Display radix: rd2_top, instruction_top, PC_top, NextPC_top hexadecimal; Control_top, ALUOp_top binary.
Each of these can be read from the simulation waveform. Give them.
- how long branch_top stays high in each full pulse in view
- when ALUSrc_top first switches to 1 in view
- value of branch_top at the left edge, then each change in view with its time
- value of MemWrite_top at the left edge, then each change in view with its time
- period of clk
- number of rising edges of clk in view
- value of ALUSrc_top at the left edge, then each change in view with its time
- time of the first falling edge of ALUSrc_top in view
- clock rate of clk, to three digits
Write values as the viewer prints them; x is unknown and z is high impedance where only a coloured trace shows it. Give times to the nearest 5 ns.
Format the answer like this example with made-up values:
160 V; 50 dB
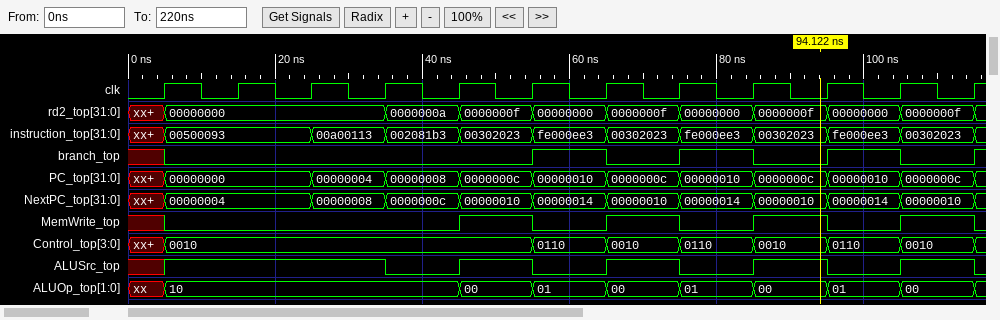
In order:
10 ns, 10 ns, 10 ns; 5 ns; x, 0 at 5 ns, 1 at 55 ns, 0 at 65 ns, 1 at 75 ns, 0 at 85 ns, 1 at 95 ns, 0 at 105 ns, 1 at 115 ns; x, 0 at 5 ns, 1 at 45 ns, 0 at 55 ns, 1 at 65 ns, 0 at 75 ns, 1 at 85 ns, 0 at 95 ns, 1 at 105 ns, 0 at 115 ns; 10 ns; 12; x, 1 at 5 ns, 0 at 35 ns, 1 at 45 ns, 0 at 55 ns, 1 at 65 ns, 0 at 75 ns, 1 at 85 ns, 0 at 95 ns, 1 at 105 ns, 0 at 115 ns; 35 ns; 100 MHz
